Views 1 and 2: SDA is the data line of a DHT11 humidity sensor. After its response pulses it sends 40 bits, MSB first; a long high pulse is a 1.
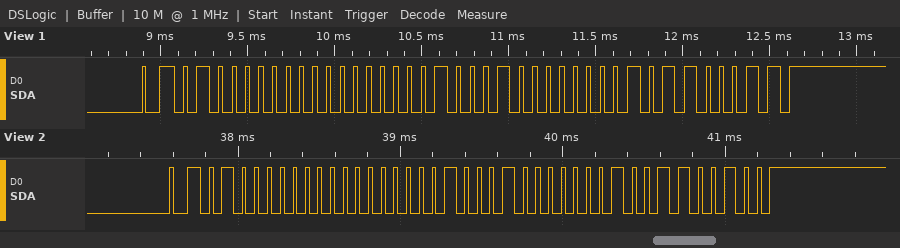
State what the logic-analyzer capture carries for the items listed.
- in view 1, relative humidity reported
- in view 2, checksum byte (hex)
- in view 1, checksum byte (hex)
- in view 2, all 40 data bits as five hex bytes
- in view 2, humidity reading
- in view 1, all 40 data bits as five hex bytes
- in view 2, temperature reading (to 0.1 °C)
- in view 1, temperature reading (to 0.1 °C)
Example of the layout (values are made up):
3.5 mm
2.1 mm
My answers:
64 %
0x64
0x63
40 00 22 02 64
64 %
40 00 22 01 63
34.2 °C
34.1 °C
